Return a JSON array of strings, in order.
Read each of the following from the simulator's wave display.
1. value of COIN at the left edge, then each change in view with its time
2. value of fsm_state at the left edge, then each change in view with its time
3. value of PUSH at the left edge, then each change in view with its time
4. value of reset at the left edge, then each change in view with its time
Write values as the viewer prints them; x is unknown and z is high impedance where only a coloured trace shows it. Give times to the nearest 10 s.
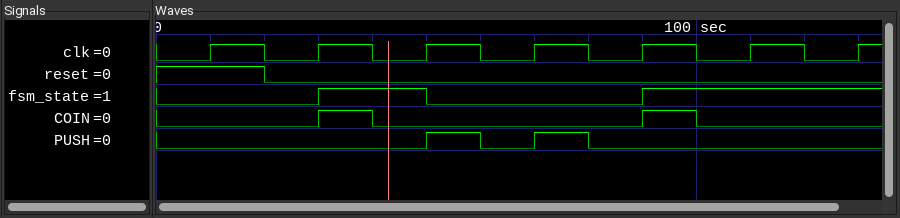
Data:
["0, 1 at 30 s, 0 at 40 s, 1 at 90 s, 0 at 100 s", "0, 1 at 30 s, 0 at 50 s, 1 at 90 s", "0, 1 at 50 s, 0 at 60 s, 1 at 70 s, 0 at 80 s", "1, 0 at 20 s"]
